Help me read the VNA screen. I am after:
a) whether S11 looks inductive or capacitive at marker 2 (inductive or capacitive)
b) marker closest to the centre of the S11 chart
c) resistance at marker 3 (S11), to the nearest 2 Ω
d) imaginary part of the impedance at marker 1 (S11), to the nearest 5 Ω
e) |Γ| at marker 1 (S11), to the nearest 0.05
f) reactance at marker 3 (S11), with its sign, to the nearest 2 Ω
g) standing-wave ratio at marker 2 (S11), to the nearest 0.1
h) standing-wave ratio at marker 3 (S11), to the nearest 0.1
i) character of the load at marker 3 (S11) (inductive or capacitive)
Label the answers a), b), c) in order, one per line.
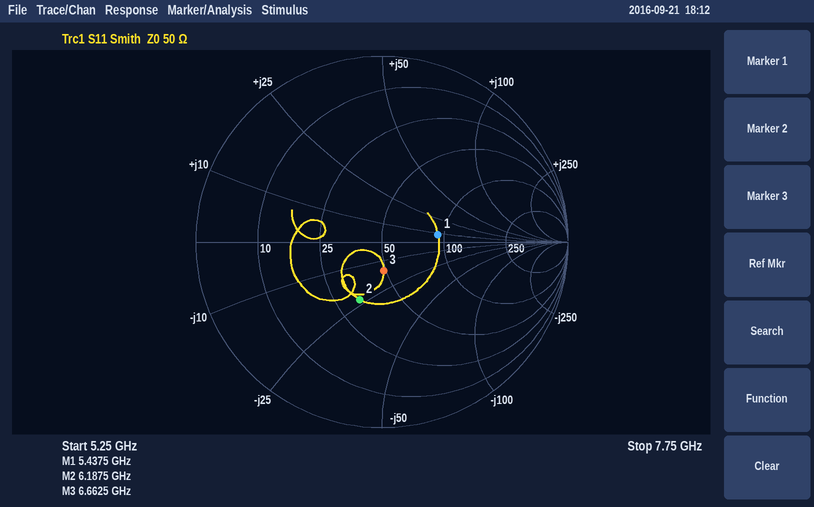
a) capacitive
b) marker 3
c) 48 Ω
d) +10 Ω
e) 0.30
f) -16 Ω
g) 2.0
h) 1.4
i) capacitive
